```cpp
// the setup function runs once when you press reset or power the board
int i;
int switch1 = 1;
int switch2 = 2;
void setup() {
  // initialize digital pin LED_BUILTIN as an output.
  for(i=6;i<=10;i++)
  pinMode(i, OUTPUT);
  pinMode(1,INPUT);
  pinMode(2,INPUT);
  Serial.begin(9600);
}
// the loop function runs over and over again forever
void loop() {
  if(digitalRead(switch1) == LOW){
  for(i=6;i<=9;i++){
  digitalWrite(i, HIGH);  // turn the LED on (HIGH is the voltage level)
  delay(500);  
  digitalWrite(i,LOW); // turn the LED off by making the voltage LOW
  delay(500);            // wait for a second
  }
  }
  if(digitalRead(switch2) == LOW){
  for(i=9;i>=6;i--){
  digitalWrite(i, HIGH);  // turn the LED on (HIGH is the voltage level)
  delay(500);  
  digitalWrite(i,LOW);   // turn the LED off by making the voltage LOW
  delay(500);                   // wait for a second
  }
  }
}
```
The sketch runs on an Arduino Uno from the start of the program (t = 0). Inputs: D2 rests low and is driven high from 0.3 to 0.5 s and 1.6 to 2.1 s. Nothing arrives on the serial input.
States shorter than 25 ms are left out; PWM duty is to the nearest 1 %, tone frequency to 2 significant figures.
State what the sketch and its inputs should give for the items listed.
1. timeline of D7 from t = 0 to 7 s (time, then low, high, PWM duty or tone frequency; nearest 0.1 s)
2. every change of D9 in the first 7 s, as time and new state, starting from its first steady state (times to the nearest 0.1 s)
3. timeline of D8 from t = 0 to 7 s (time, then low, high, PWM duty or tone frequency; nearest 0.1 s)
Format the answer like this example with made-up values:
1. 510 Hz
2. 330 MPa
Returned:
1. 0 s low; 1 s high; 1.5 s low; 6 s high; 6.5 s low
2. 0 s low; 3 s high; 3.5 s low; 4 s high; 4.5 s low
3. 0 s low; 2 s high; 2.5 s low; 5 s high; 5.5 s low
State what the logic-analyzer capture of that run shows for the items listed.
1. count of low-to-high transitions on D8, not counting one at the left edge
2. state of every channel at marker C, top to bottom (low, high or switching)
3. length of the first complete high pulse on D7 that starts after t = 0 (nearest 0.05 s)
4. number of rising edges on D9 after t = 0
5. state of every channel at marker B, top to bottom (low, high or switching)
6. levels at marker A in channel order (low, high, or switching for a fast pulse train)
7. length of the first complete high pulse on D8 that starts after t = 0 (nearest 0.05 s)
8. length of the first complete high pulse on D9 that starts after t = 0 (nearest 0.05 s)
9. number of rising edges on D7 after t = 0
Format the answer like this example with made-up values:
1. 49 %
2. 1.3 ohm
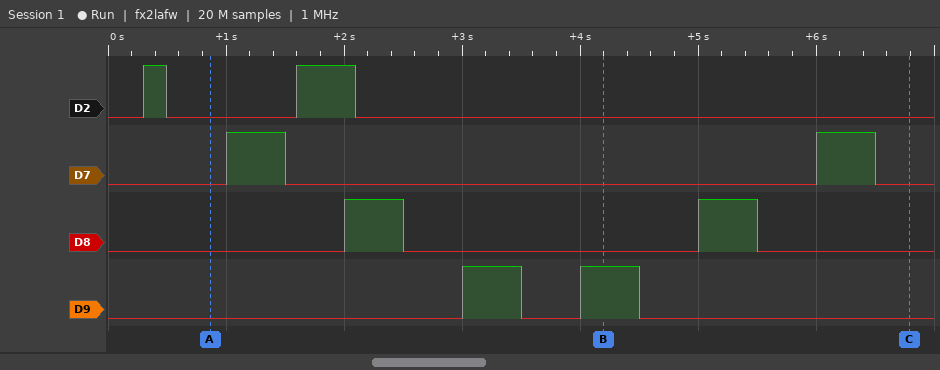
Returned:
1. 2
2. D2 low, D7 low, D8 low, D9 low
3. 0.50 s
4. 2
5. D2 low, D7 low, D8 low, D9 high
6. D2 low, D7 low, D8 low, D9 low
7. 0.50 s
8. 0.50 s
9. 2
